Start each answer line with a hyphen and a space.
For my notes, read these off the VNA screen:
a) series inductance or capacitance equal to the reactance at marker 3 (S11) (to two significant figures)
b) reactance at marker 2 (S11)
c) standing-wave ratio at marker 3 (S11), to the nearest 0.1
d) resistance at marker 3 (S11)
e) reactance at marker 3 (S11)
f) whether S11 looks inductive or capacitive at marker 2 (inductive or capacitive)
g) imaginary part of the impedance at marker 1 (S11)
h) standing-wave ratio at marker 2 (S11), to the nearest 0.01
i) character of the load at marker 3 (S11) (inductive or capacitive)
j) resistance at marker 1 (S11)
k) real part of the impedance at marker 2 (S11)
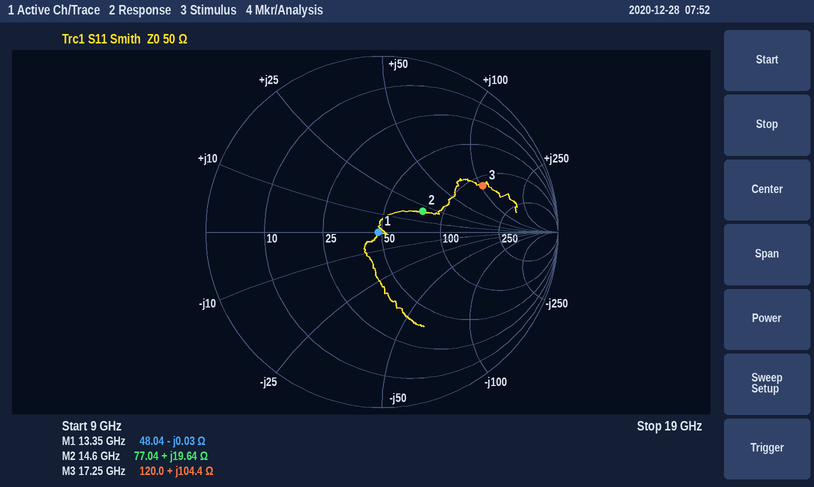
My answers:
- 960 pH
- +19.64 Ω
- 4.4
- 120.0 Ω
- +104.4 Ω
- inductive
- -0.03 Ω
- 1.70
- inductive
- 48.04 Ω
- 77.04 Ω
